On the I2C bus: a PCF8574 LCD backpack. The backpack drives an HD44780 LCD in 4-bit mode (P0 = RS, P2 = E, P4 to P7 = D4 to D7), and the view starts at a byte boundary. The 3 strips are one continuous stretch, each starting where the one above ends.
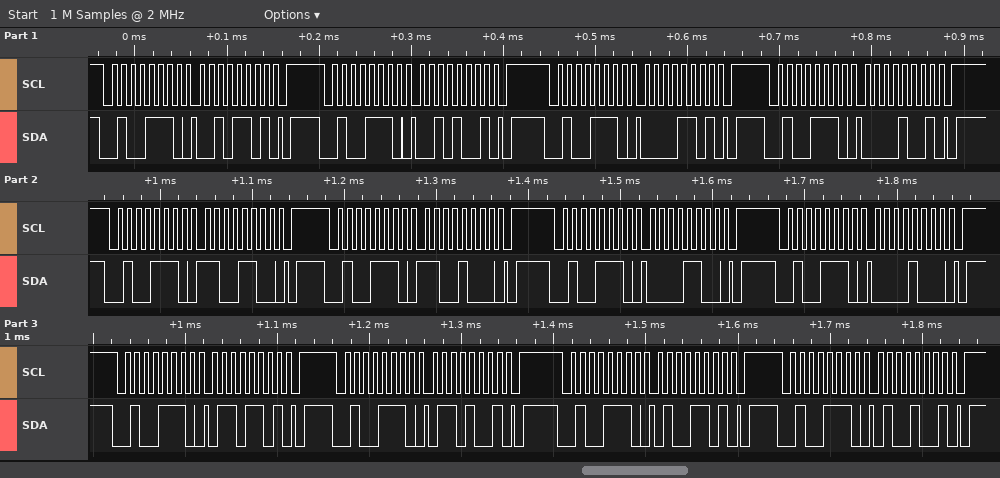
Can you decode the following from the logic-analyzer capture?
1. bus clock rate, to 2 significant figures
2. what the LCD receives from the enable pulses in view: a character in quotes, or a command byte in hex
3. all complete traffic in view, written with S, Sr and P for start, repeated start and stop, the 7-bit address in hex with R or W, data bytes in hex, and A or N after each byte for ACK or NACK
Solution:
100 kHz
' ' 0xC0 'd'
S 27W A 2D A P S 27W A 29 A P S 27W A 0D A P S 27W A 09 A P S 27W A CC A P S 27W A C8 A P S 27W A 0C A P S 27W A 08 A P S 27W A 6D A P S 27W A 69 A P S 27W A 4D A P S 27W A 49 A P
